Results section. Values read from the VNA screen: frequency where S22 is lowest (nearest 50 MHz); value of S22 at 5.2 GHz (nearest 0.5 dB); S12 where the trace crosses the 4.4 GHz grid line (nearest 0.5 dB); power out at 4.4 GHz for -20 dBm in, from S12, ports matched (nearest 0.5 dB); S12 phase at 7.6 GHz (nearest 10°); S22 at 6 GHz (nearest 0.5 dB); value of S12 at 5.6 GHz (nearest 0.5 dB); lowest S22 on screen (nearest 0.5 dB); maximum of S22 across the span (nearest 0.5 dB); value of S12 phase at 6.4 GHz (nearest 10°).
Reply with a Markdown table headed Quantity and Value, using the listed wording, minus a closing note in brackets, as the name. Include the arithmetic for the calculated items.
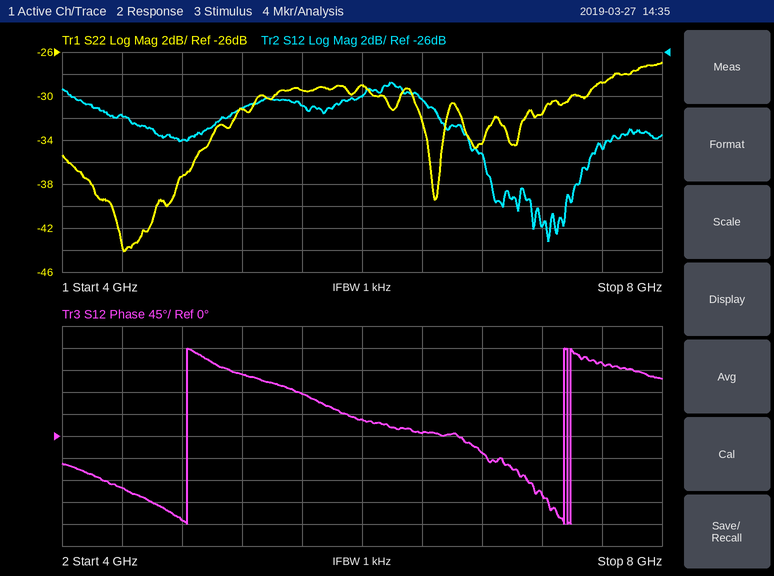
| Quantity | Value |
|---|---|
| frequency where S22 is lowest | 4.40 GHz |
| value of S22 at 5.2 GHz | -31.0 dB |
| S12 where the trace crosses the 4.4 GHz grid line | -32.0 dB |
| power out at 4.4 GHz for -20 dBm in, from S12, ports matched | -20 dBm + (-32.0 dB) = -52.0 dBm |
| S12 phase at 7.6 GHz | 150° |
| S22 at 6 GHz | -29.0 dB |
| value of S12 at 5.6 GHz | -31.0 dB |
| lowest S22 on screen | -44.0 dB |
| maximum of S22 across the span | -27.0 dB |
| value of S12 phase at 6.4 GHz | 10° |
